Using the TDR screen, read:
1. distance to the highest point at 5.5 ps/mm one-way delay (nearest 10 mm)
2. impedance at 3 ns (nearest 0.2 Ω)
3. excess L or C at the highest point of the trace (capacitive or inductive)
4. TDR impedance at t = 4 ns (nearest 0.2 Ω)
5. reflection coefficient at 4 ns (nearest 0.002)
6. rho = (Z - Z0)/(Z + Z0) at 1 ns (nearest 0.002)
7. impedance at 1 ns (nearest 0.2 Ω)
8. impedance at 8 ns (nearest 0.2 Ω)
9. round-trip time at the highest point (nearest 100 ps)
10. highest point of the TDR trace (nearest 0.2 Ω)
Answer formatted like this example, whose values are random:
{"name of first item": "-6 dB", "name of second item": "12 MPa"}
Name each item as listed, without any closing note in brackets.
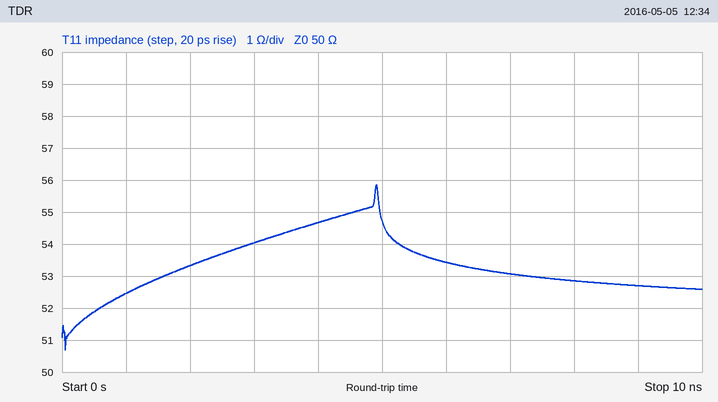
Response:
{"distance to the highest point at 5.5 ps/mm one-way delay": "450 mm", "impedance at 3 ns": "54.0 Ω", "excess L or C at the highest point of the trace": "inductive", "TDR impedance at t = 4 ns": "54.6 Ω", "reflection coefficient at 4 ns": "+0.044", "rho = (Z - Z0)/(Z + Z0) at 1 ns": "+0.024", "impedance at 1 ns": "52.4 Ω", "impedance at 8 ns": "52.8 Ω", "round-trip time at the highest point": "4.9 ns", "highest point of the TDR trace": "55.8 Ω"}
